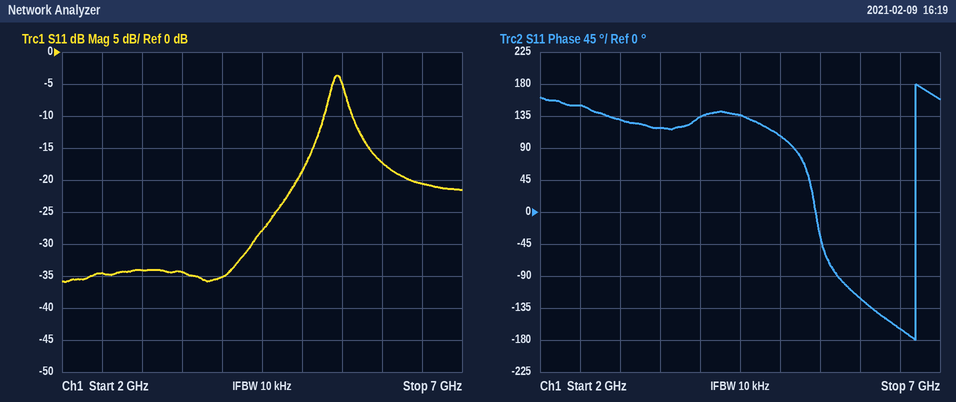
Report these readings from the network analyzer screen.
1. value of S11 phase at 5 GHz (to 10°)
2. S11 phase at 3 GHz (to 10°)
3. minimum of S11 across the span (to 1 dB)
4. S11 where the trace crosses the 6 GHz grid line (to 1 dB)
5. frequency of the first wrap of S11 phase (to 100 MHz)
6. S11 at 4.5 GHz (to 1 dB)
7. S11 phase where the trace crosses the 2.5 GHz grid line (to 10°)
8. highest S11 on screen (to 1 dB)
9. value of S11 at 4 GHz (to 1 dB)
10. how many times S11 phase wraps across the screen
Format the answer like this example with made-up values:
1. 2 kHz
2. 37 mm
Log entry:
1. 110°
2. 130°
3. -36 dB
4. -17 dB
5. 6.7 GHz
6. -28 dB
7. 150°
8. -4 dB
9. -35 dB
10. 1
